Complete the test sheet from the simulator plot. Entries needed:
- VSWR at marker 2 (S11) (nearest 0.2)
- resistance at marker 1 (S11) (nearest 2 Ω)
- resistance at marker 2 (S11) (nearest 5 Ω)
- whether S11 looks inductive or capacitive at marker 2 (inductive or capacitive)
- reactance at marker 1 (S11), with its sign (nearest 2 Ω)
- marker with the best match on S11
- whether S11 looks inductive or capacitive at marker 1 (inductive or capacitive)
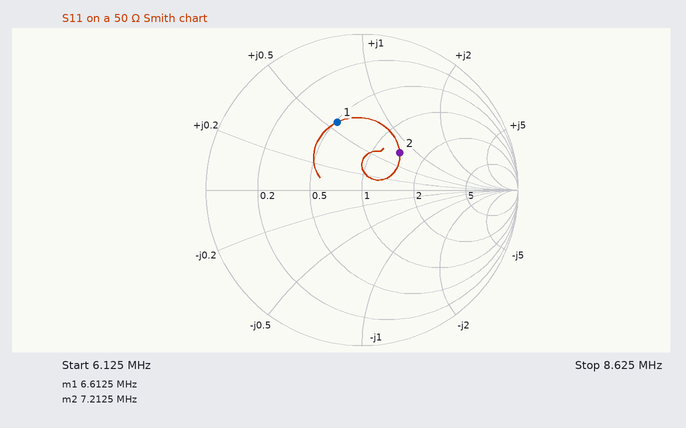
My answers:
2.0
26 Ω
70 Ω
inductive
+28 Ω
marker 2
inductive
